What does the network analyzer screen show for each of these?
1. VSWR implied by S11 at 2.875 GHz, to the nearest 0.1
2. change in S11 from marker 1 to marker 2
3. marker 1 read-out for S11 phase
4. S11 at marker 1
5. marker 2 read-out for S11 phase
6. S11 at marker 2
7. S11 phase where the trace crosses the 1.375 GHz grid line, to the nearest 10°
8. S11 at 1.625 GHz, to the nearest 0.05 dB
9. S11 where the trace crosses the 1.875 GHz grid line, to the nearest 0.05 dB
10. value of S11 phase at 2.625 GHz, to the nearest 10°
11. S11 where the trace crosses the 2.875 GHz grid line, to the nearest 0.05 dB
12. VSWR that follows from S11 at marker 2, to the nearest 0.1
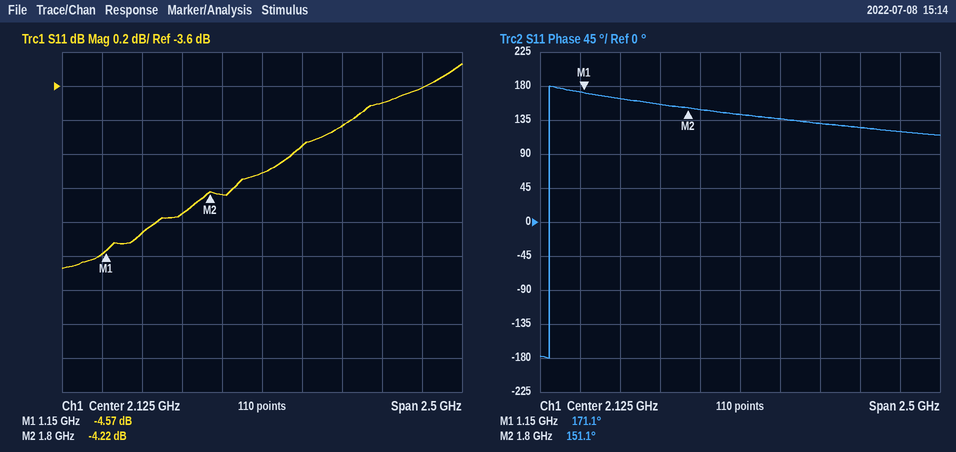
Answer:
4.8
0.35 dB
171.1°
-4.57 dB
151.1°
-4.22 dB
160°
-4.35 dB
-4.25 dB
130°
-3.70 dB
4.2
